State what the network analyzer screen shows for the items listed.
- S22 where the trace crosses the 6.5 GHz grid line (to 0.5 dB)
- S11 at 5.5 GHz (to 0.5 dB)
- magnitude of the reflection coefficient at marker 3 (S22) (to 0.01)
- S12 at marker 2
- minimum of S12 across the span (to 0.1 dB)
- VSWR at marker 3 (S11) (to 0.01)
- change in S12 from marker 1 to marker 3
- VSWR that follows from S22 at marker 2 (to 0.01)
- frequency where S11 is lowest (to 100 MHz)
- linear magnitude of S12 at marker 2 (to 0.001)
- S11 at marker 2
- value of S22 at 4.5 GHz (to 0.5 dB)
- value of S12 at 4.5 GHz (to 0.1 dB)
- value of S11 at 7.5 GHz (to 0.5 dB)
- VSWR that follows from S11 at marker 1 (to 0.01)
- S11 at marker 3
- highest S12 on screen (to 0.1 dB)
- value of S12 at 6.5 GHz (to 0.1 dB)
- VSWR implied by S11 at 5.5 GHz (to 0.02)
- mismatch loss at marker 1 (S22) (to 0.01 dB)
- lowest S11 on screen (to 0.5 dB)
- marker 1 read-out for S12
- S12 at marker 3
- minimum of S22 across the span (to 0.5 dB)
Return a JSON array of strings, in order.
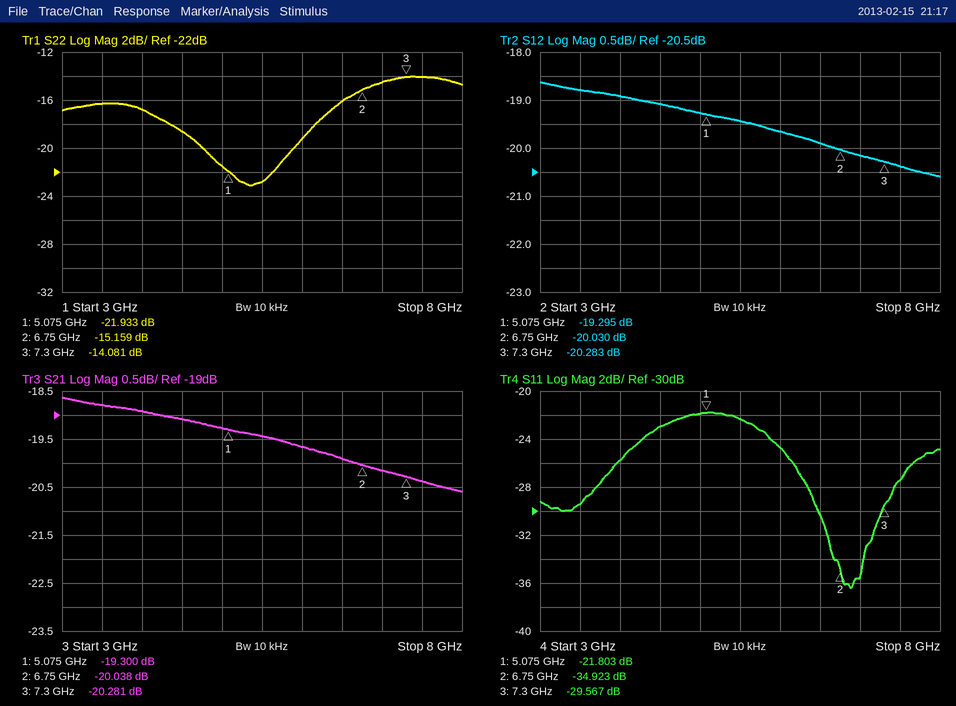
["-16.0 dB", "-22.5 dB", "0.20", "-20.030 dB", "-20.6 dB", "1.07", "-0.988 dB", "1.42", "6.9 GHz", "0.100", "-34.923 dB", "-18.5 dB", "-19.1 dB", "-27.5 dB", "1.18", "-29.567 dB", "-18.6 dB", "-19.9 dB", "1.16", "0.03 dB", "-36.5 dB", "-19.295 dB", "-20.283 dB", "-23.0 dB"]
